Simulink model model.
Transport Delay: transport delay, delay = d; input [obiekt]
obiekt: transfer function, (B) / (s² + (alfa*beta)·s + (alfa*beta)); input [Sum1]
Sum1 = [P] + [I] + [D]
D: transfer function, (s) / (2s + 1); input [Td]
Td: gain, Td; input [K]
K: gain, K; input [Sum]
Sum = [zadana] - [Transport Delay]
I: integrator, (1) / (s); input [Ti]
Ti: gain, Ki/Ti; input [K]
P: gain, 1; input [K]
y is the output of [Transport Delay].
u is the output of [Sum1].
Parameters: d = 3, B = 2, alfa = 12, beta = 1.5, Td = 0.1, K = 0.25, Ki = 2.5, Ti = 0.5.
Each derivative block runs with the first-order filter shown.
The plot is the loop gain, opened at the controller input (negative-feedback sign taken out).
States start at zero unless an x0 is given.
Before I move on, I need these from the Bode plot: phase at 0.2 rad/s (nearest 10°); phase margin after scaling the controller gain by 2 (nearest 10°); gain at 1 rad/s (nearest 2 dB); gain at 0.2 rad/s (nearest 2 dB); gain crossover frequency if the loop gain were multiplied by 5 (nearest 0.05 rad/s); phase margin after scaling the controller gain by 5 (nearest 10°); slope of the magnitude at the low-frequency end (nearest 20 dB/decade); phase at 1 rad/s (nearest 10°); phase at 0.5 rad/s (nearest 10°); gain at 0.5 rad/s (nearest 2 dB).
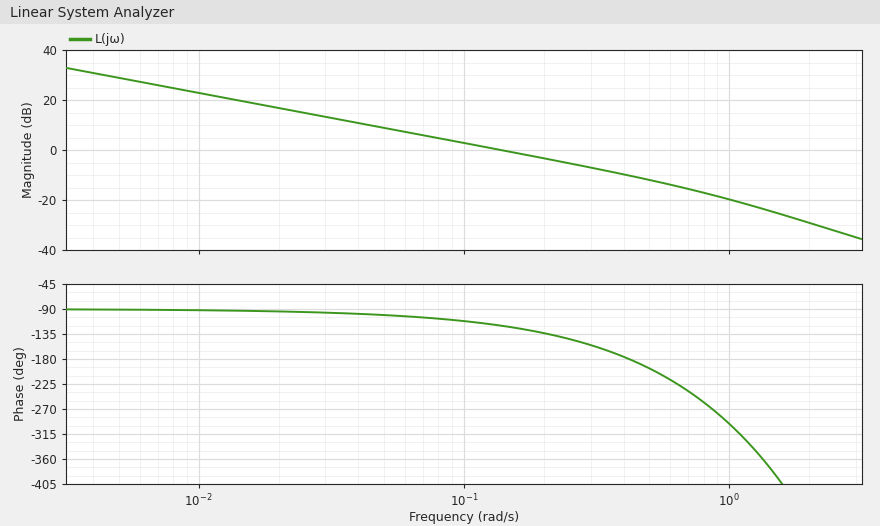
-130°
30°
-20 dB
-4 dB
0.60 rad/s
-40°
-20 dB/decade
-300°
-200°
-12 dB
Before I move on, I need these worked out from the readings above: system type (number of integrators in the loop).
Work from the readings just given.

1
